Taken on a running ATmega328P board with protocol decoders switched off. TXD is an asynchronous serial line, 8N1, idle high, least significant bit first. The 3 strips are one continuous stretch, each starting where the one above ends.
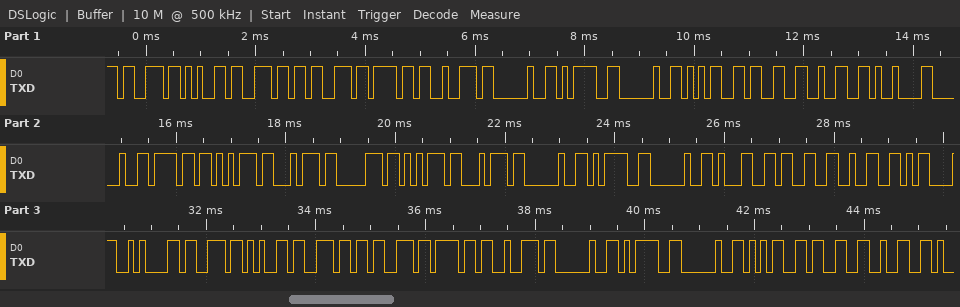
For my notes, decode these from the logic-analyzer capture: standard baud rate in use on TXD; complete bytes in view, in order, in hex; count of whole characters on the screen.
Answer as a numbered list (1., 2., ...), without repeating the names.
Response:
1. 9600 baud
2. 73 65 6E 73 6F 72 20 3D 20 35 33 32 09 20 6F 75 74 70 75 74 20 3D 20 31 33 32 0D 0A 73 65 6E 73 6F 72 20 3D 20 35 33 32
3. 40
